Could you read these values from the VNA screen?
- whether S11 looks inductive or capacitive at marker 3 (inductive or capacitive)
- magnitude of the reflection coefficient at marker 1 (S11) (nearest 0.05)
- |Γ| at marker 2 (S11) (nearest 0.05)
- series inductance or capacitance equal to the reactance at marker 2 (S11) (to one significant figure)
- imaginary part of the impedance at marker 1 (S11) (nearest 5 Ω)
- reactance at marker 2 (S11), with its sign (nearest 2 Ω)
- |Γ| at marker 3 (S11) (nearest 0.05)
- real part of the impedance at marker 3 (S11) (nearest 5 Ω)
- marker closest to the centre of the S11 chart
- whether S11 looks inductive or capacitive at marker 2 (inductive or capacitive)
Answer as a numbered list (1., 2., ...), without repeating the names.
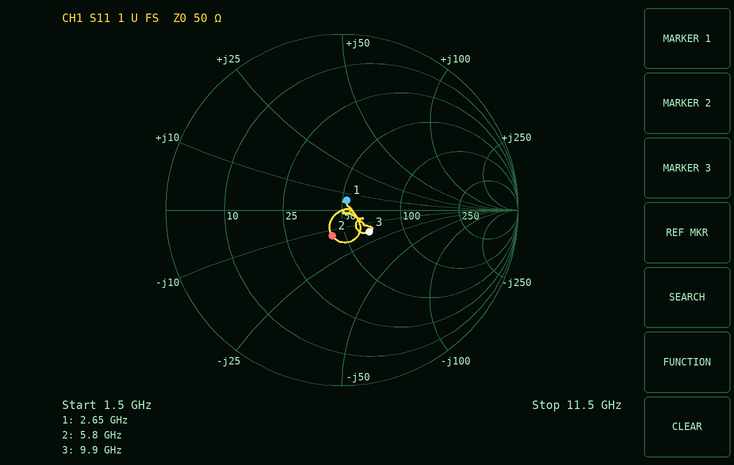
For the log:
1. capacitive
2. 0.05
3. 0.15
4. 2 pF
5. +5 Ω
6. -12 Ω
7. 0.20
8. 65 Ω
9. marker 1
10. capacitive
